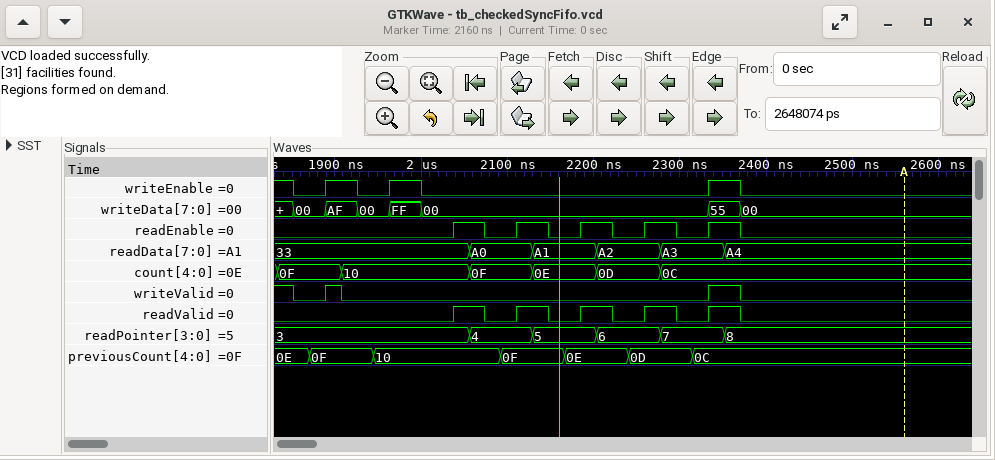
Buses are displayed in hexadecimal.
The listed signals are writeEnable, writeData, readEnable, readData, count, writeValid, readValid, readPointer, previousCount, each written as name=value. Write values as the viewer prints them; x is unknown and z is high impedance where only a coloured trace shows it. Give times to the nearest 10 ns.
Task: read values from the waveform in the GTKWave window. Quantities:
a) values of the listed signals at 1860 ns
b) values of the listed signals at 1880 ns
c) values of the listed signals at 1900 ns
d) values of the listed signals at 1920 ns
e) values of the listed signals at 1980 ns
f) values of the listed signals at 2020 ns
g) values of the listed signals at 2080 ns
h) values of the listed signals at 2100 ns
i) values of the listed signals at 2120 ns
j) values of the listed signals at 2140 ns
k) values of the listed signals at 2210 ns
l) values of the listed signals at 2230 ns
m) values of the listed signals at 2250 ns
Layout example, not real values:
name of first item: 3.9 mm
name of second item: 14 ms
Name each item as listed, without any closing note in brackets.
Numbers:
values of the listed signals at 1860 ns: writeEnable=0, writeData=00, readEnable=0, readData=33, count=0F, writeValid=0, readValid=0, readPointer=3, previousCount=0E
values of the listed signals at 1880 ns: writeEnable=0, writeData=00, readEnable=0, readData=33, count=0F, writeValid=0, readValid=0, readPointer=3, previousCount=0F
values of the listed signals at 1900 ns: writeEnable=1, writeData=AF, readEnable=0, readData=33, count=0F, writeValid=1, readValid=0, readPointer=3, previousCount=0F
values of the listed signals at 1920 ns: writeEnable=1, writeData=AF, readEnable=0, readData=33, count=10, writeValid=0, readValid=0, readPointer=3, previousCount=0F
values of the listed signals at 1980 ns: writeEnable=1, writeData=FF, readEnable=0, readData=33, count=10, writeValid=0, readValid=0, readPointer=3, previousCount=10
values of the listed signals at 2020 ns: writeEnable=0, writeData=00, readEnable=0, readData=33, count=10, writeValid=0, readValid=0, readPointer=3, previousCount=10
values of the listed signals at 2080 ns: writeEnable=0, writeData=00, readEnable=0, readData=A0, count=0F, writeValid=0, readValid=0, readPointer=4, previousCount=10
values of the listed signals at 2100 ns: writeEnable=0, writeData=00, readEnable=0, readData=A0, count=0F, writeValid=0, readValid=0, readPointer=4, previousCount=0F
values of the listed signals at 2120 ns: writeEnable=0, writeData=00, readEnable=1, readData=A0, count=0F, writeValid=0, readValid=1, readPointer=4, previousCount=0F
values of the listed signals at 2140 ns: writeEnable=0, writeData=00, readEnable=1, readData=A1, count=0E, writeValid=0, readValid=1, readPointer=5, previousCount=0F
values of the listed signals at 2210 ns: writeEnable=0, writeData=00, readEnable=1, readData=A2, count=0D, writeValid=0, readValid=1, readPointer=6, previousCount=0E
values of the listed signals at 2230 ns: writeEnable=0, writeData=00, readEnable=0, readData=A2, count=0D, writeValid=0, readValid=0, readPointer=6, previousCount=0E
values of the listed signals at 2250 ns: writeEnable=0, writeData=00, readEnable=0, readData=A2, count=0D, writeValid=0, readValid=0, readPointer=6, previousCount=0D
